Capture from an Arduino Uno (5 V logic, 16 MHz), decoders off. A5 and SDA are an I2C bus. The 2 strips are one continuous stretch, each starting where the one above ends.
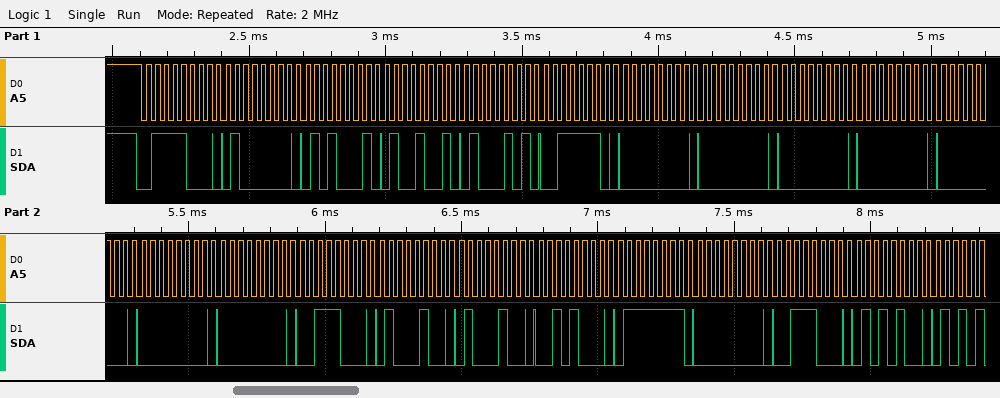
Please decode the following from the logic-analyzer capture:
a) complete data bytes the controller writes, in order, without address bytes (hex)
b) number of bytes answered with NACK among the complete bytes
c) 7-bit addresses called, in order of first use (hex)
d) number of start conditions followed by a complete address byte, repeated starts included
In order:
40 51 49 45 3E 00 00 00 00 00 00 00 38 44 44 28 7F 00 38 54
0
0x3C
1
